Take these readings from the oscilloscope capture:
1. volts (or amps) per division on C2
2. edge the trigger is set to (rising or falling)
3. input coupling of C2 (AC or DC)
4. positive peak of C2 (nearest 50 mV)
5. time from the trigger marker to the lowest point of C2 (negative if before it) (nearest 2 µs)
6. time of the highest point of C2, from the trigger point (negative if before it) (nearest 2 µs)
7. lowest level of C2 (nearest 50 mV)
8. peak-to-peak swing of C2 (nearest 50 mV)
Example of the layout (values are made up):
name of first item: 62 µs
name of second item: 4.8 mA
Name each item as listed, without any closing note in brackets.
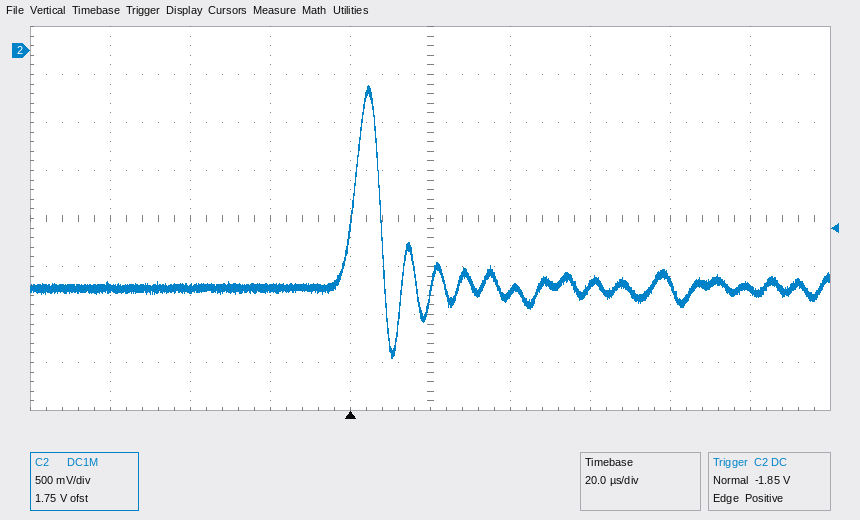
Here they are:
volts (or amps) per division on C2: 500 mV
edge the trigger is set to: rising
input coupling of C2: DC
positive peak of C2: -350 mV
time from the trigger marker to the lowest point of C2 (negative if before it): +10 µs
time of the highest point of C2, from the trigger point (negative if before it): +4 µs
lowest level of C2: -3.20 V
peak-to-peak swing of C2: 2.85 V
